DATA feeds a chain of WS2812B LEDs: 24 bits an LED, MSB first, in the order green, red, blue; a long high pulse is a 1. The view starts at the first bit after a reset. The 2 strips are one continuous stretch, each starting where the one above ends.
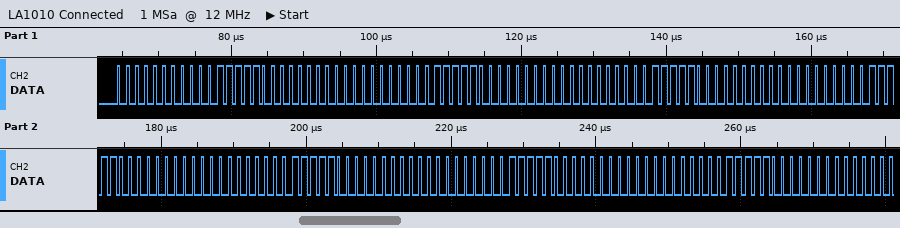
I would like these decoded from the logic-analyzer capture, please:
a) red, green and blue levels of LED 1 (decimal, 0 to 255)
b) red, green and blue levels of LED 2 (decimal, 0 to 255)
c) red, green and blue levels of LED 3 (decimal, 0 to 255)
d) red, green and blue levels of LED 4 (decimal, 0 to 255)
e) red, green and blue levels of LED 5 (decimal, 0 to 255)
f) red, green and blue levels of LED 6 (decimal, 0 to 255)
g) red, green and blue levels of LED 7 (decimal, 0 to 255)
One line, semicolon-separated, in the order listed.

31, 0, 0; 31, 0, 0; 31, 0, 0; 31, 0, 0; 31, 0, 0; 31, 0, 0; 31, 0, 0
